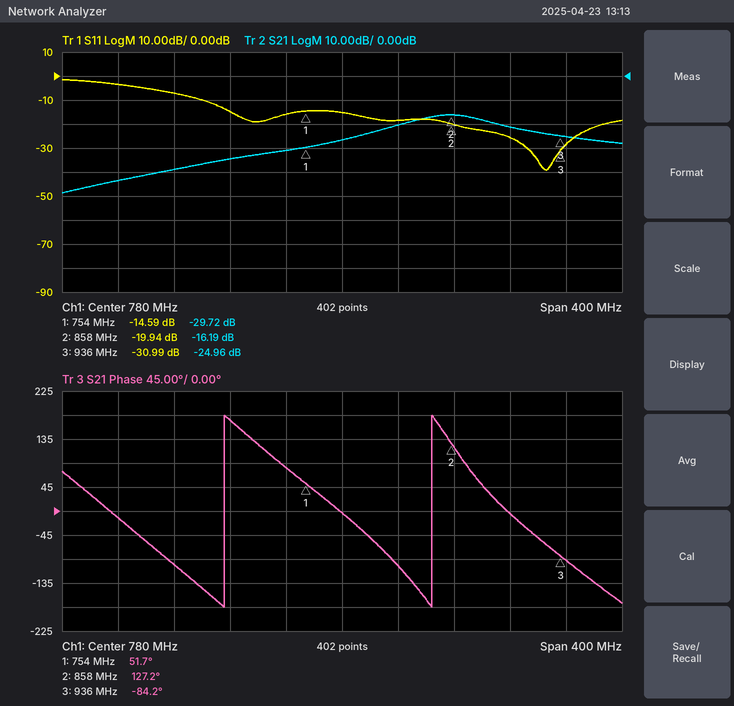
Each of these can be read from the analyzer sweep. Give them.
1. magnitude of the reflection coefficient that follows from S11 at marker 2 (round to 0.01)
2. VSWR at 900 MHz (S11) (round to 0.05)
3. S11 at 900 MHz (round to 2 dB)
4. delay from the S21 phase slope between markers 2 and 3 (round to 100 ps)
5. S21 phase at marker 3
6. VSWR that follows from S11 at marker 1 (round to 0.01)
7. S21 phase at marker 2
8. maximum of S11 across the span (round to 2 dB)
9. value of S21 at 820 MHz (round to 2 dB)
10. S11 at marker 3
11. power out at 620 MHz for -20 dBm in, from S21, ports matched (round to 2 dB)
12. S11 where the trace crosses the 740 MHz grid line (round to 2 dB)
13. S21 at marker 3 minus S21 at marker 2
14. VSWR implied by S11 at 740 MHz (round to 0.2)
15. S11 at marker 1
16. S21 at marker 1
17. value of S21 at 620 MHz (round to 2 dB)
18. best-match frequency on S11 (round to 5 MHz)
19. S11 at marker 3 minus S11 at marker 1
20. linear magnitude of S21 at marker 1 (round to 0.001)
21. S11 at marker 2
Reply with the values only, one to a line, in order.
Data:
0.10
1.10
-26 dB
7.5 ns
-84.2°
1.46
127.2°
-2 dB
-20 dB
-30.99 dB
-64 dBm
-16 dB
-8.77 dB
1.4
-14.59 dB
-29.72 dB
-44 dB
925 MHz
-16.40 dB
0.033
-19.94 dB
